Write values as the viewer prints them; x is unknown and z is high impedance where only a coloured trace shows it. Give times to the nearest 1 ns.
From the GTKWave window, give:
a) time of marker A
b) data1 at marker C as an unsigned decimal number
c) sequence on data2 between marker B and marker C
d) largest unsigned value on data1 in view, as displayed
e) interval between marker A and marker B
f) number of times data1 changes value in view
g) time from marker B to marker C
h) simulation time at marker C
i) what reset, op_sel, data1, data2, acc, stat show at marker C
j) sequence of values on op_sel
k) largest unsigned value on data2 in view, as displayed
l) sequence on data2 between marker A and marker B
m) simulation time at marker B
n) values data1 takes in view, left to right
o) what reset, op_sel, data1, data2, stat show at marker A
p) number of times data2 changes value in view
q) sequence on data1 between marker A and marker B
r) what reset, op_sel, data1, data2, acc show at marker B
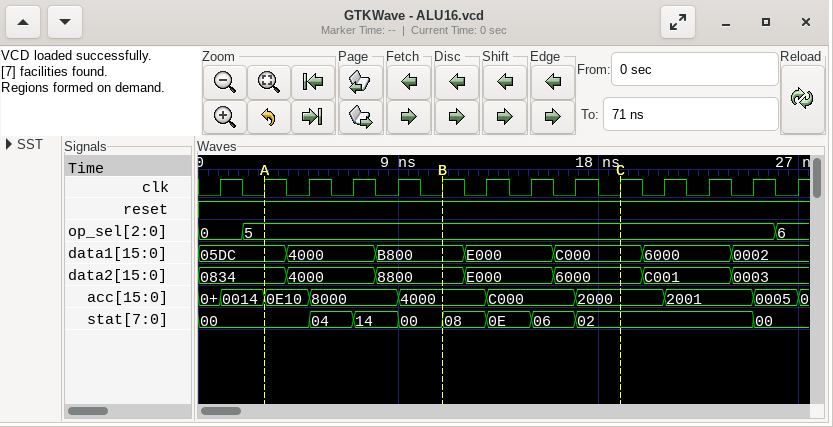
3 ns
49152
8800, E000, 6000
E000
8 ns
6
8 ns
19 ns
reset=1, op_sel=5, data1=C000, data2=6000, acc=2000, stat=02
0, 5, 6
E000
0834, 4000, 8800
11 ns
05DC, 4000, B800, E000, C000, 6000, 0002
reset=1, op_sel=5, data1=05DC, data2=0834, stat=00
6
05DC, 4000, B800
reset=1, op_sel=5, data1=B800, data2=8800, acc=4000
